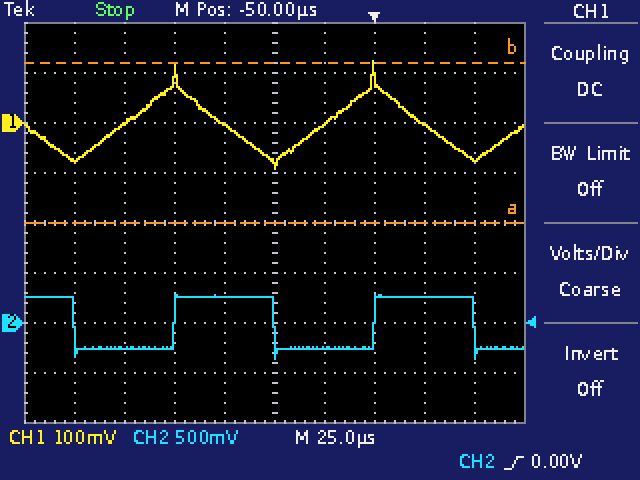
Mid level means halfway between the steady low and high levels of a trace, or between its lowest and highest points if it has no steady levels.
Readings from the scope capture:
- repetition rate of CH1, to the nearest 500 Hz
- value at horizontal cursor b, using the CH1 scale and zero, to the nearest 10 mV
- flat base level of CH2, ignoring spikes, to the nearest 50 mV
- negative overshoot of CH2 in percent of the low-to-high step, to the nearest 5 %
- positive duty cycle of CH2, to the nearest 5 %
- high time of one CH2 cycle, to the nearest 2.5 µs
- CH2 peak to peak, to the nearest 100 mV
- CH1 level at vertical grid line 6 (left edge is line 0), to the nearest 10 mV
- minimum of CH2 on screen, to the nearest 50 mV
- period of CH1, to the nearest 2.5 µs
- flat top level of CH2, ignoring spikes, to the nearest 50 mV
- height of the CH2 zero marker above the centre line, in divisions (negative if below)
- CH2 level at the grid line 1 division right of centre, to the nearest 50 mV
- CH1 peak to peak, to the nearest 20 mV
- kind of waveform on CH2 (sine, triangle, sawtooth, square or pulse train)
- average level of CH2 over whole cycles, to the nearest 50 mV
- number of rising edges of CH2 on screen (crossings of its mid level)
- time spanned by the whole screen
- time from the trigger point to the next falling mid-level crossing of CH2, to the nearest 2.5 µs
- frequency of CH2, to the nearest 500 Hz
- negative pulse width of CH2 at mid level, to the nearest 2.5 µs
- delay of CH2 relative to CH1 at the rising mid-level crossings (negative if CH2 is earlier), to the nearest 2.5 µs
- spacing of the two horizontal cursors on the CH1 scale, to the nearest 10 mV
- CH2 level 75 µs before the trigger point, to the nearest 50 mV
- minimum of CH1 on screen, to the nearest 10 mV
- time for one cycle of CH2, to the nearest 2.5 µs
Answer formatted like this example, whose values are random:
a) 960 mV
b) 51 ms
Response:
a) 10.0 kHz
b) 120 mV
c) -250 mV
d) 20 %
e) 50 %
f) 50.0 µs
g) 600 mV
h) 0 mV
i) -350 mV
j) 100.0 µs
k) 250 mV
l) -2.0 div
m) -250 mV
n) 220 mV
o) square
p) 0 mV
q) 2
r) 250 µs
s) 50.0 µs
t) 10.0 kHz
u) 50.0 µs
v) +17.5 µs
w) 320 mV
x) 250 mV
y) -90 mV
z) 100.0 µs
